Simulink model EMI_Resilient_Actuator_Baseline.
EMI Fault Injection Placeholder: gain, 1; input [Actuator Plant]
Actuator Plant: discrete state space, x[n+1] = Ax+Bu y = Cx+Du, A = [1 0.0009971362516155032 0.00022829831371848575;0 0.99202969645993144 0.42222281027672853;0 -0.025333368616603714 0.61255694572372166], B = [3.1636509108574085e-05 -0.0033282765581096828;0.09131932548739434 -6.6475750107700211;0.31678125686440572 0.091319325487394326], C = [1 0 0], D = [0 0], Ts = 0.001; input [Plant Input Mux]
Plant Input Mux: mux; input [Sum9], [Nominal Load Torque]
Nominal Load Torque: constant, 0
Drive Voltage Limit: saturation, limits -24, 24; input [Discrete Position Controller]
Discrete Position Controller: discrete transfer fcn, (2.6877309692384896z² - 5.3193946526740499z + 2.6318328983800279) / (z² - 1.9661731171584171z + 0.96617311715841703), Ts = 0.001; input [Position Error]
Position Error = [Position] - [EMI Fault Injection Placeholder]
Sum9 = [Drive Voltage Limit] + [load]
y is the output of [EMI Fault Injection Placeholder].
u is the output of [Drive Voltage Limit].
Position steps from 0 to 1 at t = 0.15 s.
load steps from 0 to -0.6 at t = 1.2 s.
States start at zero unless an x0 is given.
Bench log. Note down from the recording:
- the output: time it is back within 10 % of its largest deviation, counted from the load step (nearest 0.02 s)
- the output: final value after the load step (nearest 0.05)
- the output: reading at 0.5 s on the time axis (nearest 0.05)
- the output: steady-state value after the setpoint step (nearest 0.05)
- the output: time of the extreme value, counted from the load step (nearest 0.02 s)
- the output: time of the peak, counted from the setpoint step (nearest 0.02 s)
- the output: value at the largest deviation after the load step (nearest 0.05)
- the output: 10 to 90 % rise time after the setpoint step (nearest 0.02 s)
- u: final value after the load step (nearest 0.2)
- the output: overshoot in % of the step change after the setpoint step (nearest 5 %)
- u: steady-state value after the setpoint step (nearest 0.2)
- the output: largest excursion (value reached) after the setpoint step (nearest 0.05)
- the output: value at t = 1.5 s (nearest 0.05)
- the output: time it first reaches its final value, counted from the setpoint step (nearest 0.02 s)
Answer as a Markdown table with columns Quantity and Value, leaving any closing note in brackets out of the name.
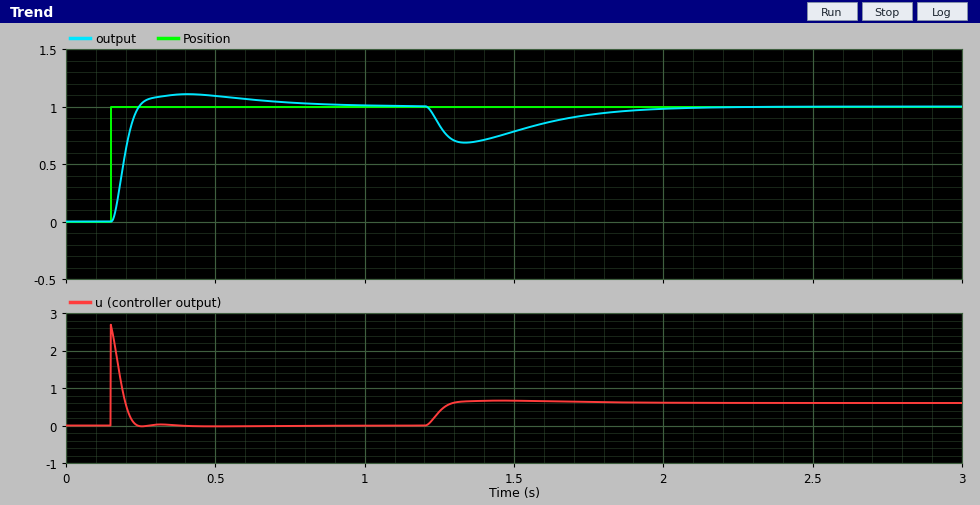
| Quantity | Value |
|---|---|
| the output: time it is back within 10 % of its largest deviation, counted from the load step | 0.72 s |
| the output: final value after the load step | 1.00 |
| the output: reading at 0.5 s on the time axis | 1.10 |
| the output: steady-state value after the setpoint step | 1.00 |
| the output: time of the extreme value, counted from the load step | 0.14 s |
| the output: time of the peak, counted from the setpoint step | 0.26 s |
| the output: value at the largest deviation after the load step | 0.70 |
| the output: 10 to 90 % rise time after the setpoint step | 0.06 s |
| u: final value after the load step | 0.6 |
| the output: overshoot in % of the step change after the setpoint step | 10 % |
| u: steady-state value after the setpoint step | 0.0 |
| the output: largest excursion (value reached) after the setpoint step | 1.10 |
| the output: value at t = 1.5 s | 0.80 |
| the output: time it first reaches its final value, counted from the setpoint step | 0.10 s |
